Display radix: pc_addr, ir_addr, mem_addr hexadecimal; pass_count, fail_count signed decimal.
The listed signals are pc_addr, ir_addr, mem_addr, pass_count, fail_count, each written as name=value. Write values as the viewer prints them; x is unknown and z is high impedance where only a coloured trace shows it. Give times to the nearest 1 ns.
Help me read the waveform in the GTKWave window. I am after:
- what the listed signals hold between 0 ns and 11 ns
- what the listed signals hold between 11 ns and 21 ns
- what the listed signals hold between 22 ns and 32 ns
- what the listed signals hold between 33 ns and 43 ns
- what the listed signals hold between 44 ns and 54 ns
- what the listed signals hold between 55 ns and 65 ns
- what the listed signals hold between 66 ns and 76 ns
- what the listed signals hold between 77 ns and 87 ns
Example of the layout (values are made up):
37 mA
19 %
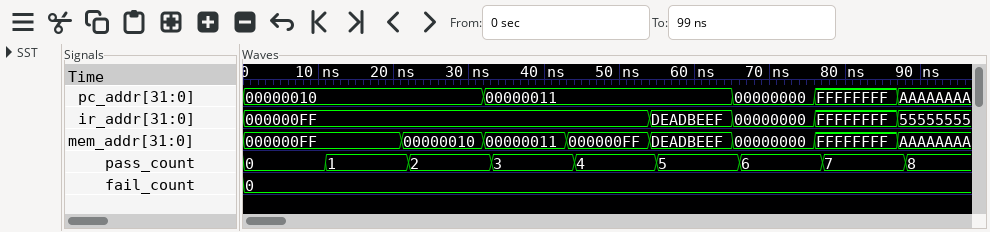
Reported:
pc_addr=00000010, ir_addr=000000FF, mem_addr=000000FF, pass_count=0, fail_count=0
pc_addr=00000010, ir_addr=000000FF, mem_addr=000000FF, pass_count=1, fail_count=0
pc_addr=00000010, ir_addr=000000FF, mem_addr=00000010, pass_count=2, fail_count=0
pc_addr=00000011, ir_addr=000000FF, mem_addr=00000011, pass_count=3, fail_count=0
pc_addr=00000011, ir_addr=000000FF, mem_addr=000000FF, pass_count=4, fail_count=0
pc_addr=00000011, ir_addr=DEADBEEF, mem_addr=DEADBEEF, pass_count=5, fail_count=0
pc_addr=00000000, ir_addr=00000000, mem_addr=00000000, pass_count=6, fail_count=0
pc_addr=FFFFFFFF, ir_addr=FFFFFFFF, mem_addr=FFFFFFFF, pass_count=7, fail_count=0
